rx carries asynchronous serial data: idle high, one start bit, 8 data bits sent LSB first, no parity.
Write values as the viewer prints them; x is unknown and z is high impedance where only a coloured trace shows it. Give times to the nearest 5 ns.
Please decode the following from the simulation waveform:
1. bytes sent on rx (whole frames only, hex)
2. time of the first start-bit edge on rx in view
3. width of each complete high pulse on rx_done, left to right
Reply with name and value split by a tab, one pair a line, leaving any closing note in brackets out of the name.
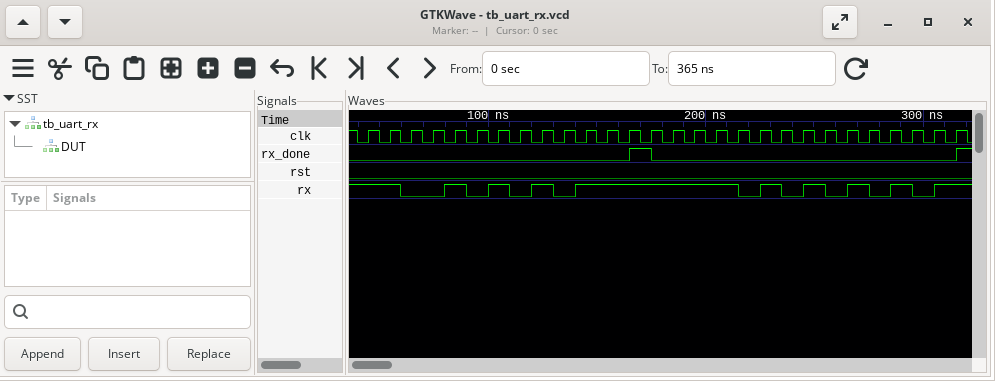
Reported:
bytes sent on rx	AA, 55
time of the first start-bit edge on rx in view	60 ns
width of each complete high pulse on rx_done, left to right	10 ns
